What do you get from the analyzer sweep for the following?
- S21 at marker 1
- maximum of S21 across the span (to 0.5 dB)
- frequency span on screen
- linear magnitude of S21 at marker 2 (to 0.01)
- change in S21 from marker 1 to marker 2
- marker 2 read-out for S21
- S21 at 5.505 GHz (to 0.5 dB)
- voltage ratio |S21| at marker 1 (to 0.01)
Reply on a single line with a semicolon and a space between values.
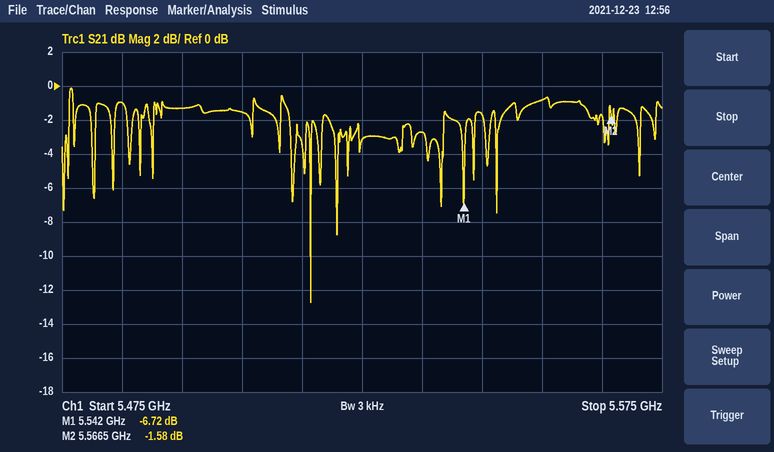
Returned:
-6.72 dB; 0.0 dB; 100 MHz; 0.83; 5.14 dB; -1.58 dB; -1.5 dB; 0.46
